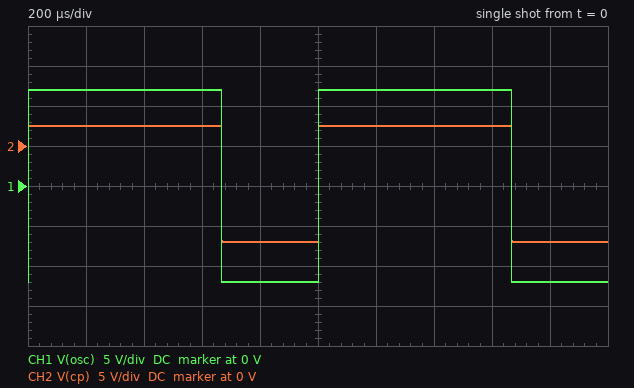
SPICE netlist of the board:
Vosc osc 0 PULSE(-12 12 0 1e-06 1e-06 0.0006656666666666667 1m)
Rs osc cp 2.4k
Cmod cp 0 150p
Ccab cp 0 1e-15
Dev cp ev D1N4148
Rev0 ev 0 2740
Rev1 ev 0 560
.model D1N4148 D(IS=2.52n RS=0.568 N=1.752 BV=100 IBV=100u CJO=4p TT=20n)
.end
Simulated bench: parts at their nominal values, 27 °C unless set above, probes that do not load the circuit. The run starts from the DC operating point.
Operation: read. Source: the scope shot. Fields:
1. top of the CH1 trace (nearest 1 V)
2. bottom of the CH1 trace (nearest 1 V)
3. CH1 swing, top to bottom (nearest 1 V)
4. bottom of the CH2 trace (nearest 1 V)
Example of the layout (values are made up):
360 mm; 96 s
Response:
12 V; -12 V; 24 V; -12 V
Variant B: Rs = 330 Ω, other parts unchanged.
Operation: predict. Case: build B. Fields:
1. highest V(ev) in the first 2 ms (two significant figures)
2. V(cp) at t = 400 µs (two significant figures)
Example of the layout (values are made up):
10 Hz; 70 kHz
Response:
6.6 V; 7.3 V
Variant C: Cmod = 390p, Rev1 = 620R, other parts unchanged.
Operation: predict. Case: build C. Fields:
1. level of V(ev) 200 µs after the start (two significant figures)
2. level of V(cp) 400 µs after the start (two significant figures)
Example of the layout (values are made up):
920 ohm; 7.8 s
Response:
2.0 V; 2.6 V
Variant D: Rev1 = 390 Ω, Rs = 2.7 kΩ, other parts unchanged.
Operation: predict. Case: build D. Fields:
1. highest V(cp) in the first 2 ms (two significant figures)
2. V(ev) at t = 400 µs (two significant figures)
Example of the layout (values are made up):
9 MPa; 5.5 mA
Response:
1.9 V; 1.3 V
